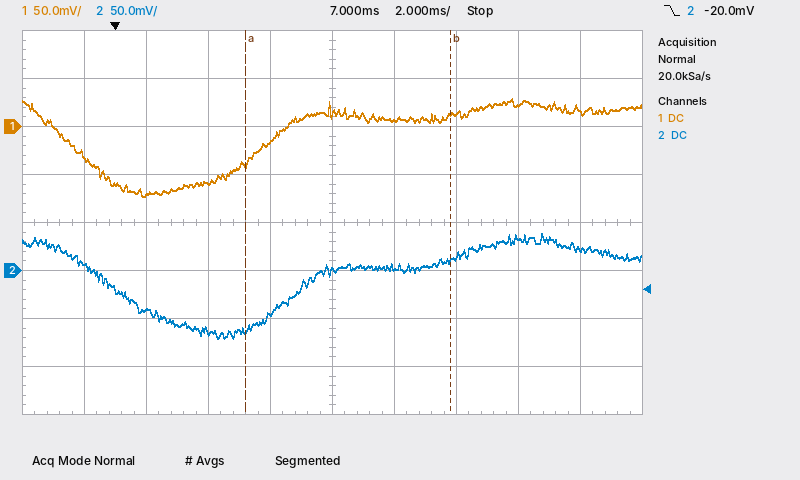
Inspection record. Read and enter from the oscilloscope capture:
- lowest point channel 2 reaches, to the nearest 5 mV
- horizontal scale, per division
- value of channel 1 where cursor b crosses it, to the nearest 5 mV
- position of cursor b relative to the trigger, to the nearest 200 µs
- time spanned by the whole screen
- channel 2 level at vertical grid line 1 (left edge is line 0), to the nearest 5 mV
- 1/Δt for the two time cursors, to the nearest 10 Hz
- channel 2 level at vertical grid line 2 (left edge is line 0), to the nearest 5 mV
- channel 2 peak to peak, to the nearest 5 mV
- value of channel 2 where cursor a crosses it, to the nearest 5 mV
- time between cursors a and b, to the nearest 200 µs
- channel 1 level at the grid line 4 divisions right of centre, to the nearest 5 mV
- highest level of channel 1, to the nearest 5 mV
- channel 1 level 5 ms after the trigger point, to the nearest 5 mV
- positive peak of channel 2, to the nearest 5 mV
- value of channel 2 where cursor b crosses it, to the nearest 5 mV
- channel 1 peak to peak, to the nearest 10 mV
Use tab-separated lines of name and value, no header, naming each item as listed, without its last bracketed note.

lowest point channel 2 reaches, to the nearest 5 mV	-70 mV
horizontal scale, per division	2 ms
value of channel 1 where cursor b crosses it, to the nearest 5 mV	10 mV
position of cursor b relative to the trigger, to the nearest 200 µs	+10.8 ms
time spanned by the whole screen	20 ms
channel 2 level at vertical grid line 1 (left edge is line 0), to the nearest 5 mV	5 mV
1/Δt for the two time cursors, to the nearest 10 Hz	150 Hz
channel 2 level at vertical grid line 2 (left edge is line 0), to the nearest 5 mV	-40 mV
channel 2 peak to peak, to the nearest 5 mV	110 mV
value of channel 2 where cursor a crosses it, to the nearest 5 mV	-60 mV
time between cursors a and b, to the nearest 200 µs	6.6 ms
channel 1 level at the grid line 4 divisions right of centre, to the nearest 5 mV	15 mV
highest level of channel 1, to the nearest 5 mV	30 mV
channel 1 level 5 ms after the trigger point, to the nearest 5 mV	-15 mV
positive peak of channel 2, to the nearest 5 mV	40 mV
value of channel 2 where cursor b crosses it, to the nearest 5 mV	10 mV
channel 1 peak to peak, to the nearest 10 mV	100 mV
